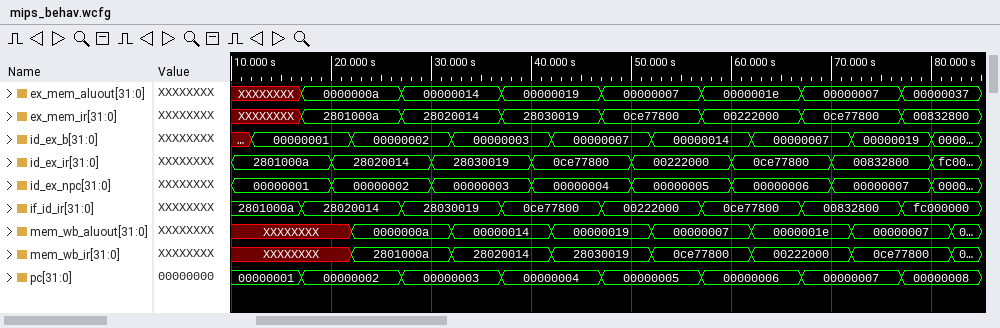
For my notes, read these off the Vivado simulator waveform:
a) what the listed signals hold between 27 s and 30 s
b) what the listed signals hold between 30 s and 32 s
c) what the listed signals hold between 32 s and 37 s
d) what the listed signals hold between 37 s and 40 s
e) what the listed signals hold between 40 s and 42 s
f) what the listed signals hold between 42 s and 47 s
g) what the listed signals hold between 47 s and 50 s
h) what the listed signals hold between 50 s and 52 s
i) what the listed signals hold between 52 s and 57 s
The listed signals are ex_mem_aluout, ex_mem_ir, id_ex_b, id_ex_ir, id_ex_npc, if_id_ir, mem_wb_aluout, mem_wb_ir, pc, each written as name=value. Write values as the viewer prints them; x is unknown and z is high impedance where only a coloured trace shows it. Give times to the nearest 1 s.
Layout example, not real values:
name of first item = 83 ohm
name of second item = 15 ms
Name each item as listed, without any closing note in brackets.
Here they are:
what the listed signals hold between 27 s and 30 s = ex_mem_aluout=00000014, ex_mem_ir=28020014, id_ex_b=00000002, id_ex_ir=28020014, id_ex_npc=00000002, if_id_ir=28030019, mem_wb_aluout=0000000a, mem_wb_ir=2801000a, pc=00000003
what the listed signals hold between 30 s and 32 s = ex_mem_aluout=00000014, ex_mem_ir=28020014, id_ex_b=00000002, id_ex_ir=28030019, id_ex_npc=00000003, if_id_ir=28030019, mem_wb_aluout=0000000a, mem_wb_ir=2801000a, pc=00000003
what the listed signals hold between 32 s and 37 s = ex_mem_aluout=00000014, ex_mem_ir=28020014, id_ex_b=00000003, id_ex_ir=28030019, id_ex_npc=00000003, if_id_ir=28030019, mem_wb_aluout=00000014, mem_wb_ir=28020014, pc=00000003
what the listed signals hold between 37 s and 40 s = ex_mem_aluout=00000019, ex_mem_ir=28030019, id_ex_b=00000003, id_ex_ir=28030019, id_ex_npc=00000003, if_id_ir=0ce77800, mem_wb_aluout=00000014, mem_wb_ir=28020014, pc=00000004
what the listed signals hold between 40 s and 42 s = ex_mem_aluout=00000019, ex_mem_ir=28030019, id_ex_b=00000003, id_ex_ir=0ce77800, id_ex_npc=00000004, if_id_ir=0ce77800, mem_wb_aluout=00000014, mem_wb_ir=28020014, pc=00000004
what the listed signals hold between 42 s and 47 s = ex_mem_aluout=00000019, ex_mem_ir=28030019, id_ex_b=00000007, id_ex_ir=0ce77800, id_ex_npc=00000004, if_id_ir=0ce77800, mem_wb_aluout=00000019, mem_wb_ir=28030019, pc=00000004
what the listed signals hold between 47 s and 50 s = ex_mem_aluout=00000007, ex_mem_ir=0ce77800, id_ex_b=00000007, id_ex_ir=0ce77800, id_ex_npc=00000004, if_id_ir=00222000, mem_wb_aluout=00000019, mem_wb_ir=28030019, pc=00000005
what the listed signals hold between 50 s and 52 s = ex_mem_aluout=00000007, ex_mem_ir=0ce77800, id_ex_b=00000007, id_ex_ir=00222000, id_ex_npc=00000005, if_id_ir=00222000, mem_wb_aluout=00000019, mem_wb_ir=28030019, pc=00000005
what the listed signals hold between 52 s and 57 s = ex_mem_aluout=00000007, ex_mem_ir=0ce77800, id_ex_b=00000014, id_ex_ir=00222000, id_ex_npc=00000005, if_id_ir=00222000, mem_wb_aluout=00000007, mem_wb_ir=0ce77800, pc=00000005
